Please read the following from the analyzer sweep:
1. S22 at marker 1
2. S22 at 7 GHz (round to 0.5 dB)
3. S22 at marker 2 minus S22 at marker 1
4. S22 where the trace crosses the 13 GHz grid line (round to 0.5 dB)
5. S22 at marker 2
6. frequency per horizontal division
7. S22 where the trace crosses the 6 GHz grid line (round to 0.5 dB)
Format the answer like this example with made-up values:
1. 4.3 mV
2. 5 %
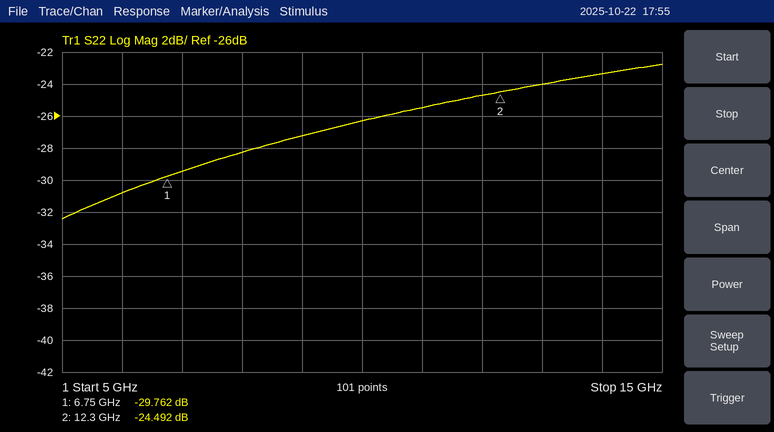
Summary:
1. -29.762 dB
2. -29.5 dB
3. 5.270 dB
4. -24.0 dB
5. -24.492 dB
6. 1 GHz
7. -31.0 dB
